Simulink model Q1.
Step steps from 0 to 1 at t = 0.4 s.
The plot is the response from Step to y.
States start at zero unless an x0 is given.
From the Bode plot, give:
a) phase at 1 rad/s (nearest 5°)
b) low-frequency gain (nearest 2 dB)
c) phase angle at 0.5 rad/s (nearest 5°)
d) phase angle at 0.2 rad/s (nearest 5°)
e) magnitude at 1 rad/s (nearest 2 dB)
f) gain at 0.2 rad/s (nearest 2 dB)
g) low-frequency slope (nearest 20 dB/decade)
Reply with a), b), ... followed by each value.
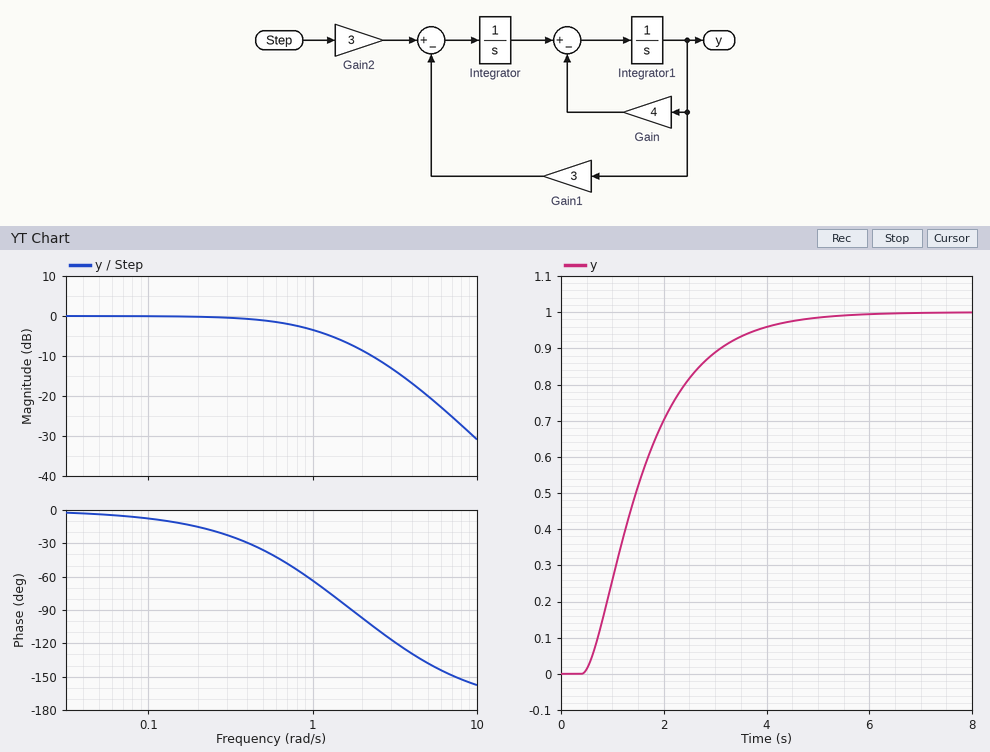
a) -65°
b) 0 dB
c) -35°
d) -15°
e) -4 dB
f) 0 dB
g) 0 dB/decade
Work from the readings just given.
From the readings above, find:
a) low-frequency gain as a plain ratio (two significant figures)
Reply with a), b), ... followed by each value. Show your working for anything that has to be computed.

a) 10^(0 / 20) = 1.0
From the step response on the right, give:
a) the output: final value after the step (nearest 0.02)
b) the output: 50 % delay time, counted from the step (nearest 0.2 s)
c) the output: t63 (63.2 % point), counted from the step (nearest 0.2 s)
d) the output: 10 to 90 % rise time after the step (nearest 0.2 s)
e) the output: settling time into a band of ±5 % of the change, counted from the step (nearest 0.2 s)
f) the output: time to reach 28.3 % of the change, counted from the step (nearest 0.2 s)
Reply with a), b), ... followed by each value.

a) 1.00
b) 1.0 s
c) 1.4 s
d) 2.4 s
e) 3.4 s
f) 0.6 s
